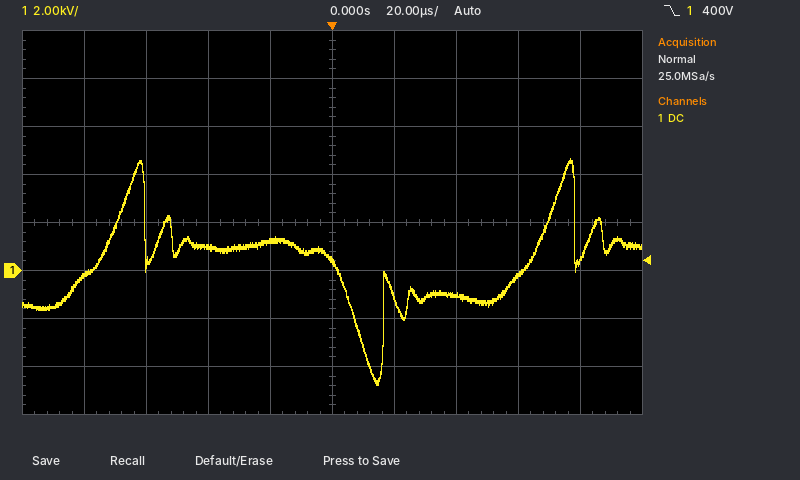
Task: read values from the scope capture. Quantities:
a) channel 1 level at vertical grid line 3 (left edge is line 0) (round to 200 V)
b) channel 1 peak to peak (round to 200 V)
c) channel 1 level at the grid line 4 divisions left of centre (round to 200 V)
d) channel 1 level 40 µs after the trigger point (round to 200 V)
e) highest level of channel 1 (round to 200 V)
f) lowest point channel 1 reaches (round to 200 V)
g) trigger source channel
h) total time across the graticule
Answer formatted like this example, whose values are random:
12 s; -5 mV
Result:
1.0 kV; 9.4 kV; -200 V; -1.0 kV; 4.6 kV; -4.8 kV; channel 1; 200 µs
